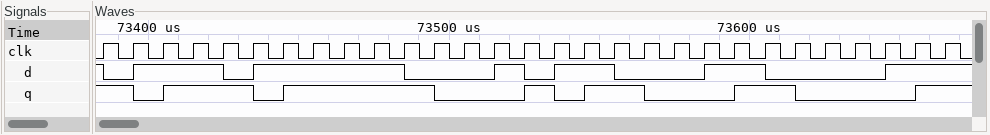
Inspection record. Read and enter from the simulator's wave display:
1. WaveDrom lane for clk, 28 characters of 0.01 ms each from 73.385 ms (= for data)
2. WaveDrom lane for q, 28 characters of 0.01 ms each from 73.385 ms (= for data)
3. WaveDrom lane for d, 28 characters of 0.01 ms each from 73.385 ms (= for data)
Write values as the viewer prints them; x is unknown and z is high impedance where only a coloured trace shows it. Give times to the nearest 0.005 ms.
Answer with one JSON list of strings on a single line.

["{name: 'clk', wave: 'p...........................'}", "{name: 'q', wave: '101..01....0..101.0..1.0...1'}", "{name: 'd', wave: '01..01....0..101.0..1.0...1.'}"]
